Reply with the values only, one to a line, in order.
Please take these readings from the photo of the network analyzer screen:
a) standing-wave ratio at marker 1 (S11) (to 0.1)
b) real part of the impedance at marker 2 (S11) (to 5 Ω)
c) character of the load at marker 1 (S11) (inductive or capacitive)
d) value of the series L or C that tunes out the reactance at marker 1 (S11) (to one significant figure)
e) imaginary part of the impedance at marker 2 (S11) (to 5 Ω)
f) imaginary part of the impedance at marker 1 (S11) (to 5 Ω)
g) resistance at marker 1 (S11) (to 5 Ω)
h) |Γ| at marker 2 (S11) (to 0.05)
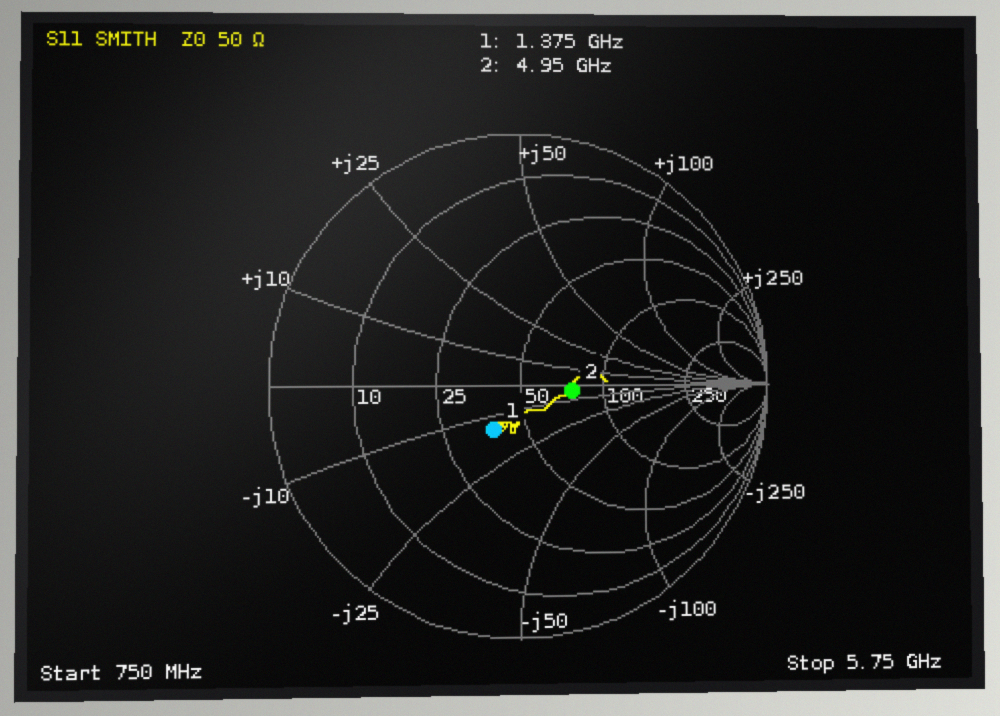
1.5
75 Ω
capacitive
2 nH
-5 Ω
-15 Ω
40 Ω
0.20
